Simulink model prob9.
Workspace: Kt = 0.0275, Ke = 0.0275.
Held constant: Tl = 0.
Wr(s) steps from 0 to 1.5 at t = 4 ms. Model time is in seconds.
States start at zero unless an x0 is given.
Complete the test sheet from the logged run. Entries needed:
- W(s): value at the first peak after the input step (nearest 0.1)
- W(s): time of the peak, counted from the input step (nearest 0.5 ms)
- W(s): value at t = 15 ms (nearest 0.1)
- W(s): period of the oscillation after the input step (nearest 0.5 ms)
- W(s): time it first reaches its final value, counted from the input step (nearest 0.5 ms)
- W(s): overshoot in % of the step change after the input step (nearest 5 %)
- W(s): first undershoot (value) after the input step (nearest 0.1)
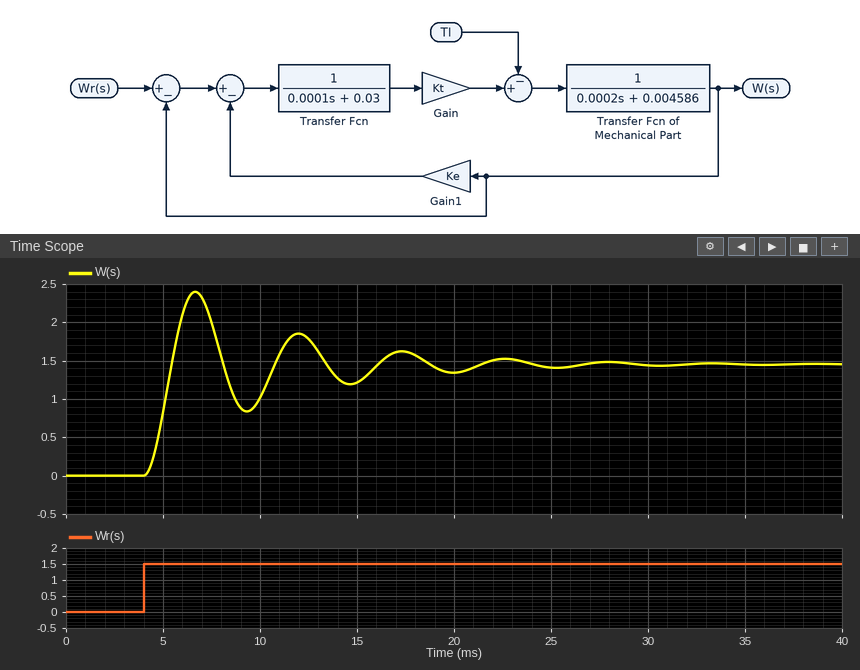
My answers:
2.4
2.5 ms
1.2
5.5 ms
1.5 ms
65 %
0.8
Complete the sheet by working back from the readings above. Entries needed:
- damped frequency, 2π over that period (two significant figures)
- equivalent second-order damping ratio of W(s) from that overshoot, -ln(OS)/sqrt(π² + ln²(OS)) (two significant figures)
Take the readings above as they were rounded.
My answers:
1.1 rad/ms
0.14
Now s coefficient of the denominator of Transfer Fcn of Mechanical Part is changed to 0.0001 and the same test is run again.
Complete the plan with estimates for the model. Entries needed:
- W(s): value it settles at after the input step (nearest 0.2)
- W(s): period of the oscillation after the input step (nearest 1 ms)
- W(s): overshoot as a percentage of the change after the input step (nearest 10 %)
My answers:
1.4
4 ms
70 %
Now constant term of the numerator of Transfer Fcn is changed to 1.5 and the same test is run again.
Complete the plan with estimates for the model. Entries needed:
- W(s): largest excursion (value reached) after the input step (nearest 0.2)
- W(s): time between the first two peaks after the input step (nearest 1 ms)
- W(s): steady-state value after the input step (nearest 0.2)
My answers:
2.4
4 ms
1.4
